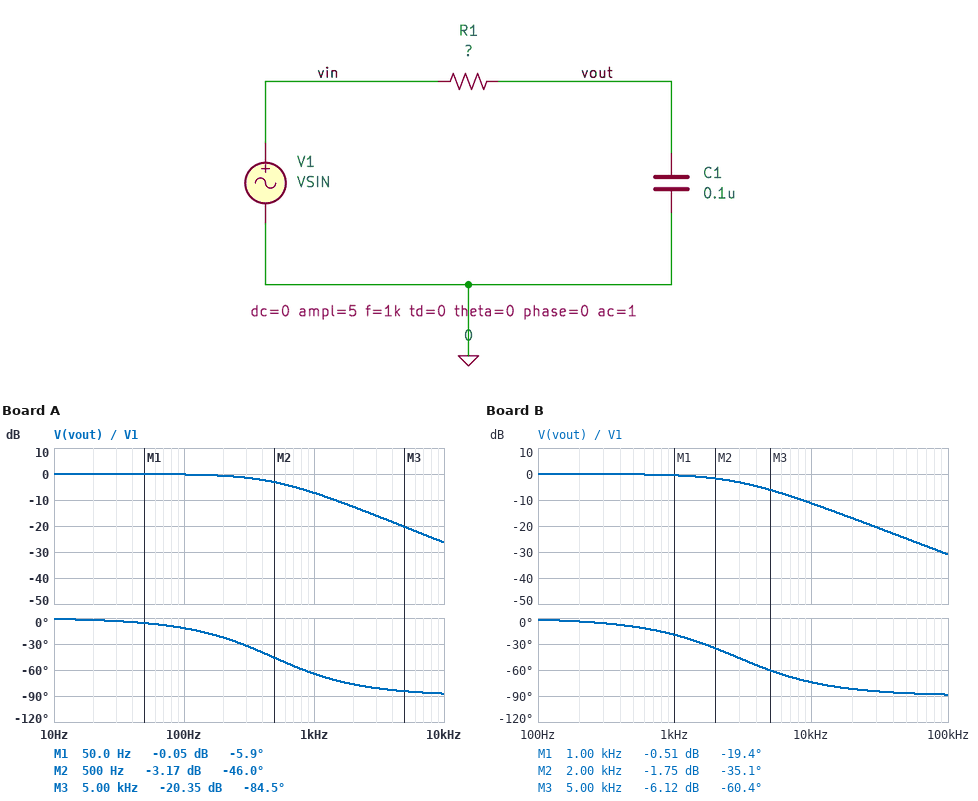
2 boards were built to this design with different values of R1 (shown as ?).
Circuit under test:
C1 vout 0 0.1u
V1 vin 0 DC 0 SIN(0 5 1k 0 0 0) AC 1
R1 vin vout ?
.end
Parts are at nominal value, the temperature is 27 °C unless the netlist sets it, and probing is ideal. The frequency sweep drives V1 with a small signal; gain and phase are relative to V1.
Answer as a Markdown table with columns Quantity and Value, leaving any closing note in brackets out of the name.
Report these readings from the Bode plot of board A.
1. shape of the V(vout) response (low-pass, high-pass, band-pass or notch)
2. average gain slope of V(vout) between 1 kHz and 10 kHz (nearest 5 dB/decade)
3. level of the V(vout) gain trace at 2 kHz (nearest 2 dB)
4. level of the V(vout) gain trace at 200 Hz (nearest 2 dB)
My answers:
| Quantity | Value |
|---|---|
| shape of the V(vout) response | low-pass |
| average gain slope of V(vout) between 1 kHz and 10 kHz | -20 dB/decade |
| level of the V(vout) gain trace at 2 kHz | -12 dB |
| level of the V(vout) gain trace at 200 Hz | 0 dB |
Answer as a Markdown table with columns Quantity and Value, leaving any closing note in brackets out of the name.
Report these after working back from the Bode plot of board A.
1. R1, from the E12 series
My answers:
| Quantity | Value |
|---|---|
| R1, from the E12 series | 3.3 kΩ |
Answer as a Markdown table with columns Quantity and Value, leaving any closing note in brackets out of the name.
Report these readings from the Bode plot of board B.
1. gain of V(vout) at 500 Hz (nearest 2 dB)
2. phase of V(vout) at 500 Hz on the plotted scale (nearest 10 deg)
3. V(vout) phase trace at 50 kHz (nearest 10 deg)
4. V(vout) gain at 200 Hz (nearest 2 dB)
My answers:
| Quantity | Value |
|---|---|
| gain of V(vout) at 500 Hz | 0 dB |
| phase of V(vout) at 500 Hz on the plotted scale | -10 deg |
| V(vout) phase trace at 50 kHz | -90 deg |
| V(vout) gain at 200 Hz | 0 dB |
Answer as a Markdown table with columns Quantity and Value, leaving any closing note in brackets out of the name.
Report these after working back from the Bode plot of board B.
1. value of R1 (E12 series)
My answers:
| Quantity | Value |
|---|---|
| value of R1 | 560 Ω |
